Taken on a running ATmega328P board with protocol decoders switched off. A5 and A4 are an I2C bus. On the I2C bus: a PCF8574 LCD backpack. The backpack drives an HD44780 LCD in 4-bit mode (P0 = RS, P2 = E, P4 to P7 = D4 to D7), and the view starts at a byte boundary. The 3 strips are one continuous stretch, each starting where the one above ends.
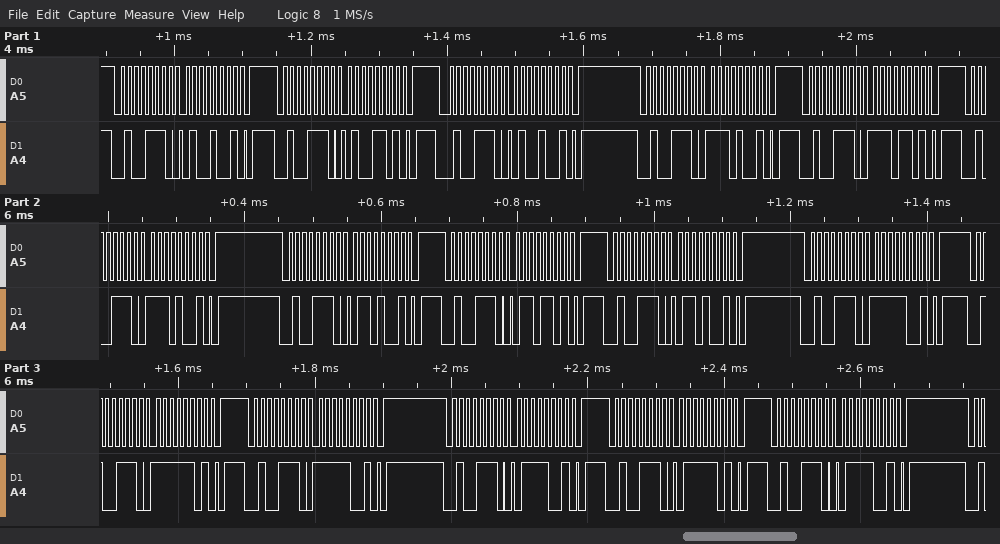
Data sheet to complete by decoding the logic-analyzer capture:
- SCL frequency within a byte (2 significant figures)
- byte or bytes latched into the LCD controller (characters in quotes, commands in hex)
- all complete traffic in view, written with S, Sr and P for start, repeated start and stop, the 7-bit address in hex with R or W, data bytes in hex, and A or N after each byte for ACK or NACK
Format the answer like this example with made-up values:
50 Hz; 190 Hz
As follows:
100 kHz; 'N' 'o'; S 27W A 49 A P S 27W A 4D A P S 27W A 49 A P S 27W A E9 A P S 27W A ED A P S 27W A E9 A P S 27W A 69 A P S 27W A 6D A P S 27W A 69 A P S 27W A F9 A P S 27W A FD A P S 27W A F9 A P S 27W A 79 A P S 27W A 7D A P S 27W A 79 A P
